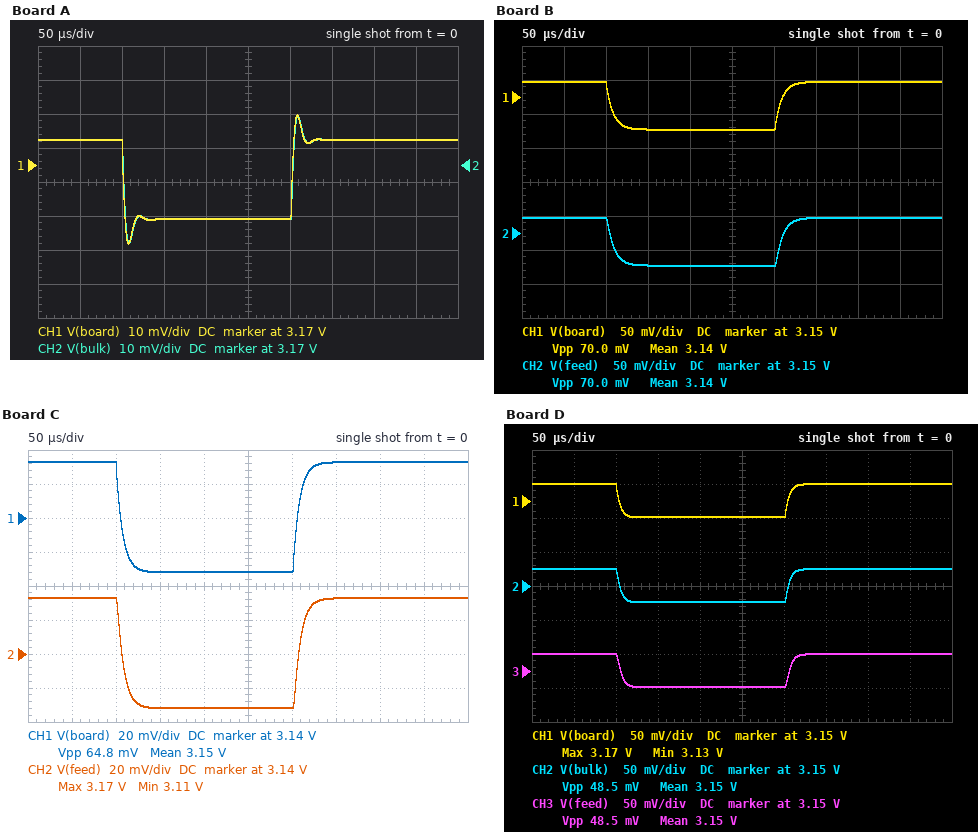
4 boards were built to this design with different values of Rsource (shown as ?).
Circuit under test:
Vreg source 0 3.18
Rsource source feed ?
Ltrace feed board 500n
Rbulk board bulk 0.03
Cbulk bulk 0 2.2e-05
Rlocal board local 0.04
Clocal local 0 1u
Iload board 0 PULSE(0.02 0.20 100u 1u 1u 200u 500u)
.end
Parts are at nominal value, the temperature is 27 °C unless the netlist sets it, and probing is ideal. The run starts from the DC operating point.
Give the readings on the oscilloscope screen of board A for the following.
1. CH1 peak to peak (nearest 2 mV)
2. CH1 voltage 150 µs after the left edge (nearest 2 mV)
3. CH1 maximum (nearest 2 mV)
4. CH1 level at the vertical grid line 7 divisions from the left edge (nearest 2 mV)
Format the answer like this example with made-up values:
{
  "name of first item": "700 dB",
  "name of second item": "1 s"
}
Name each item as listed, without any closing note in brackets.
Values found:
{
  "CH1 peak to peak": "38 mV",
  "CH1 voltage 150 µs after the left edge": "3.154 V",
  "CH1 maximum": "3.184 V",
  "CH1 level at the vertical grid line 7 divisions from the left edge": "3.178 V"
}
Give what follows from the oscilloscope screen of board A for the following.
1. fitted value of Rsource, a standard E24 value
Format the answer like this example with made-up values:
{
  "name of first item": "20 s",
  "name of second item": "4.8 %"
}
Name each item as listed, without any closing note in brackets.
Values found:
{
  "fitted value of Rsource, a standard E24 value": "0.13 Ω"
}
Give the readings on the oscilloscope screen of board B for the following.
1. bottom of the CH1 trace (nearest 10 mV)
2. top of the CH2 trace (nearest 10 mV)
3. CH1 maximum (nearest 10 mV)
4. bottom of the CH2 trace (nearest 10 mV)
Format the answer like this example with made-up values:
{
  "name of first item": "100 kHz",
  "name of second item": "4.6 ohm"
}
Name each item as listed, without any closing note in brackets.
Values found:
{
  "bottom of the CH1 trace": "3.10 V",
  "top of the CH2 trace": "3.17 V",
  "CH1 maximum": "3.17 V",
  "bottom of the CH2 trace": "3.10 V"
}
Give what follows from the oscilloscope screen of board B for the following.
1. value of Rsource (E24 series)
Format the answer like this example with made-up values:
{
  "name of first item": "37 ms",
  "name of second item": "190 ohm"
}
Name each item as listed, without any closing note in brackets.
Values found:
{
  "value of Rsource": "0.39 Ω"
}
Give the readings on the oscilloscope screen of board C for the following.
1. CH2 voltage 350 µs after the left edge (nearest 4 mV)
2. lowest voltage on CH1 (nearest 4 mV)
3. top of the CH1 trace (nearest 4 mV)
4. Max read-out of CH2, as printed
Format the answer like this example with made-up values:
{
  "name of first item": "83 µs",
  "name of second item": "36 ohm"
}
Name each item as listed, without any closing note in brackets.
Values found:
{
  "CH2 voltage 350 µs after the left edge": "3.172 V",
  "lowest voltage on CH1": "3.108 V",
  "top of the CH1 trace": "3.172 V",
  "Max read-out of CH2, as printed": "3.17 V"
}
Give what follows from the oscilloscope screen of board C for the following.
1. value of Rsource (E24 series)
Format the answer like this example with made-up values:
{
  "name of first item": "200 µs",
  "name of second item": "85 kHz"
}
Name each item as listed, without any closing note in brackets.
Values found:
{
  "value of Rsource": "0.36 Ω"
}
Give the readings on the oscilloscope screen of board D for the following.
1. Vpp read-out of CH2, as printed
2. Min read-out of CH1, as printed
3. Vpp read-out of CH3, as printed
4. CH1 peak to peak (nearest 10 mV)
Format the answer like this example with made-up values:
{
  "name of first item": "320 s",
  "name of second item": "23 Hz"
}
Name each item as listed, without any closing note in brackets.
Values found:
{
  "Vpp read-out of CH2, as printed": "48.5 mV",
  "Min read-out of CH1, as printed": "3.13 V",
  "Vpp read-out of CH3, as printed": "48.5 mV",
  "CH1 peak to peak": "50 mV"
}
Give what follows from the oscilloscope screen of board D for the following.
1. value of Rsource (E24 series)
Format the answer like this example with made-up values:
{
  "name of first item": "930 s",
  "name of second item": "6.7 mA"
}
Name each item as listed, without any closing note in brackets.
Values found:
{
  "value of Rsource": "0.27 Ω"
}
